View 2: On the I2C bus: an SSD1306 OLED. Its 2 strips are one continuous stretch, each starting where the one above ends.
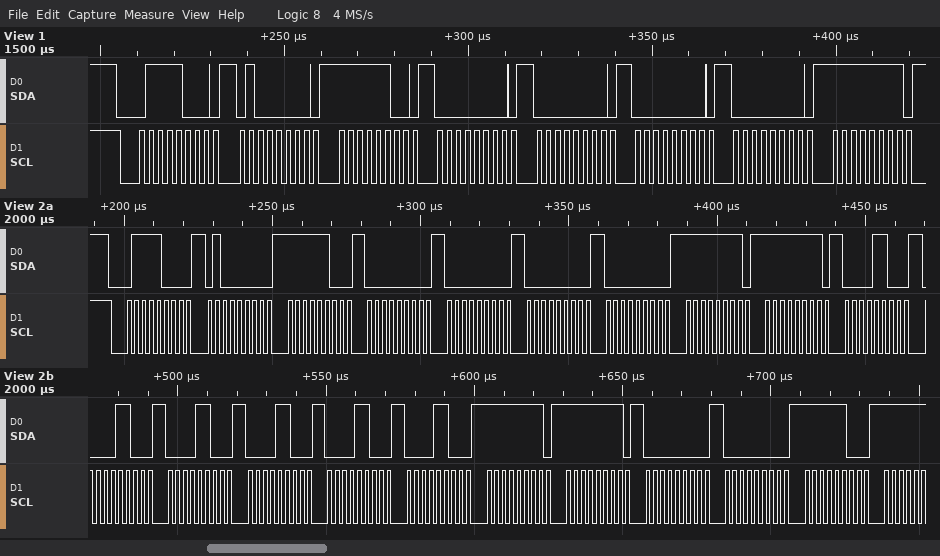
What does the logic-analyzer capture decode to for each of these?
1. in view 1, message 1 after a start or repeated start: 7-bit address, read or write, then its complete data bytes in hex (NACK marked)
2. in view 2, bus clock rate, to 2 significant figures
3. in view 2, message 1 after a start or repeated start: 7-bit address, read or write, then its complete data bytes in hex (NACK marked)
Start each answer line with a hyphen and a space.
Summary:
- 0x3C write: 40 FC 00 00 00 00 FF
- 400 kHz
- 0x3C write: 40 FC 00 00 00 00 FF FF 0C 0C 0C 0C 0C 0C FF FF 00 00 FC
